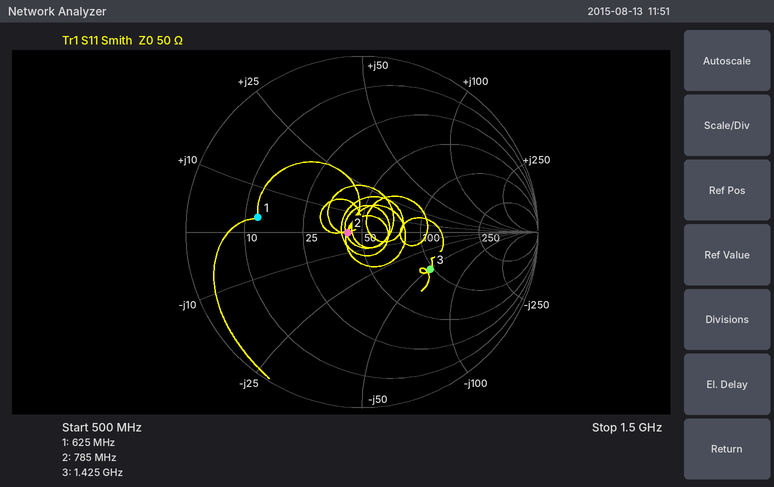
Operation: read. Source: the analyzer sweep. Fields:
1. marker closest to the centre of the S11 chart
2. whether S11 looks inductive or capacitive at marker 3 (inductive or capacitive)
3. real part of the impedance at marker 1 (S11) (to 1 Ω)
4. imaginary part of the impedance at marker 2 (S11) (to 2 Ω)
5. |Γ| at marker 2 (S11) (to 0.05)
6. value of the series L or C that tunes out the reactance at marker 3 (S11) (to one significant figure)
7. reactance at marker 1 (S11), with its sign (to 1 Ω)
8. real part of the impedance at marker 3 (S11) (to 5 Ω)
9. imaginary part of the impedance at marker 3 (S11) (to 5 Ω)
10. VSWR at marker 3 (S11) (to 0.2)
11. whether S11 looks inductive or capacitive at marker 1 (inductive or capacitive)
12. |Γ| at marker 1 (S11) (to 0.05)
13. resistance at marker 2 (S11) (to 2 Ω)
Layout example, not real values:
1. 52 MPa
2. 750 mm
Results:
1. marker 2
2. capacitive
3. 13 Ω
4. 0 Ω
5. 0.10
6. 6 nH
7. +3 Ω
8. 95 Ω
9. -50 Ω
10. 2.6
11. inductive
12. 0.60
13. 42 Ω
